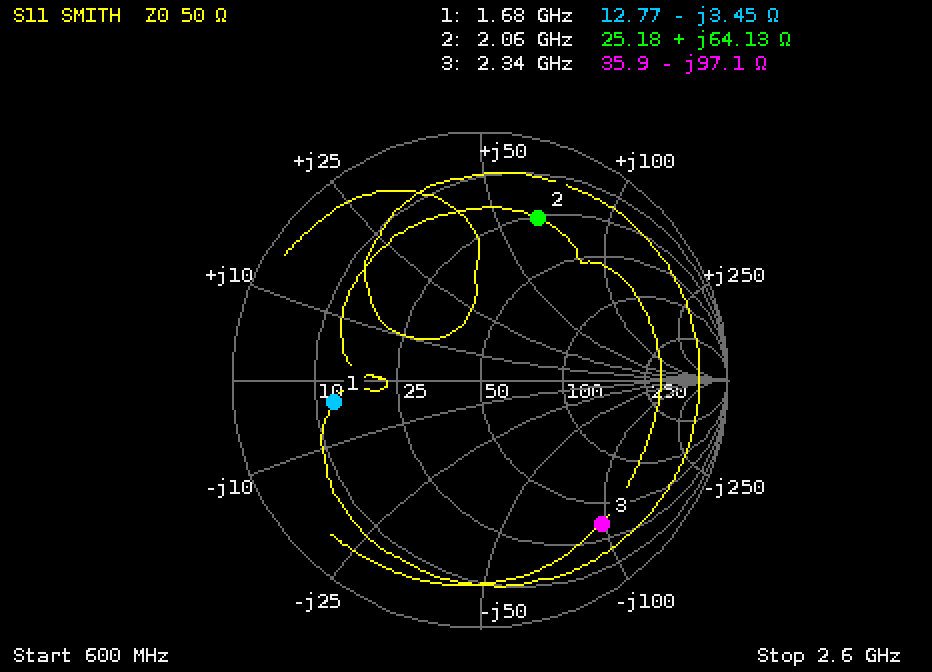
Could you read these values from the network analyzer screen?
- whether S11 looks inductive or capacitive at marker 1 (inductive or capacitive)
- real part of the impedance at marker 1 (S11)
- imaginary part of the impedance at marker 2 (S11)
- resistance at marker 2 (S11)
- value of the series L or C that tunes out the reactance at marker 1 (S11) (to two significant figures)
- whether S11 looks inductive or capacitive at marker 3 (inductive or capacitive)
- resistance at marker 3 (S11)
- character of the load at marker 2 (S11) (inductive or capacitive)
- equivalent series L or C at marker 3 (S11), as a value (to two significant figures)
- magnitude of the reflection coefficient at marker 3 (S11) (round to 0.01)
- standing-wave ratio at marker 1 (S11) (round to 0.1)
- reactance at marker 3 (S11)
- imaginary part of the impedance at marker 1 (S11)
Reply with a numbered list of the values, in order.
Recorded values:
1. capacitive
2. 12.77 Ω
3. +64.13 Ω
4. 25.18 Ω
5. 330 pH
6. capacitive
7. 35.9 Ω
8. inductive
9. 700 fF
10. 0.76
11. 3.9
12. -97.1 Ω
13. -3.45 Ω
